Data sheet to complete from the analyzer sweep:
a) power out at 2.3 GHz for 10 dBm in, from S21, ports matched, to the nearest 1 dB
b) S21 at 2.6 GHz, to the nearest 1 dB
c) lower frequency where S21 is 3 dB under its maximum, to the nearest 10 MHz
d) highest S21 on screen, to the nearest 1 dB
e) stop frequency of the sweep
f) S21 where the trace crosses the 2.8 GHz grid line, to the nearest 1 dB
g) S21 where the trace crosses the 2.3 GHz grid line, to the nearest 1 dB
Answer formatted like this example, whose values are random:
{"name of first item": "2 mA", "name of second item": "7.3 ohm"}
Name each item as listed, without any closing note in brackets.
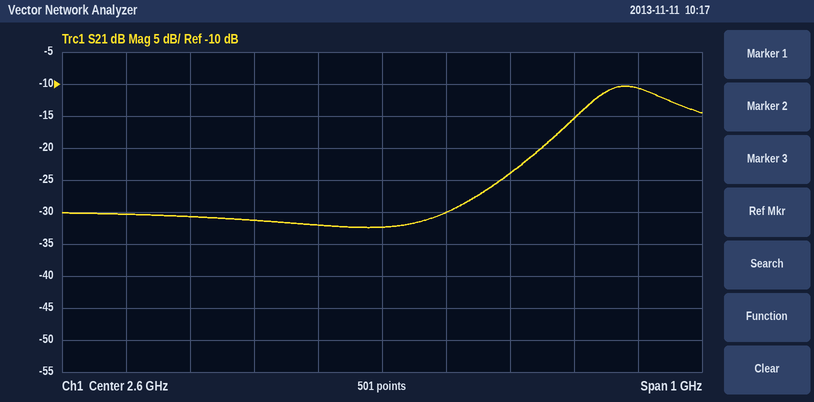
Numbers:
{"power out at 2.3 GHz for 10 dBm in, from S21, ports matched, to the nearest 1 dB": "-21 dBm", "S21 at 2.6 GHz, to the nearest 1 dB": "-32 dB", "lower frequency where S21 is 3 dB under its maximum, to the nearest 10 MHz": "2.92 GHz", "highest S21 on screen, to the nearest 1 dB": "-10 dB", "stop frequency of the sweep": "3.1 GHz", "S21 where the trace crosses the 2.8 GHz grid line, to the nearest 1 dB": "-24 dB", "S21 where the trace crosses the 2.3 GHz grid line, to the nearest 1 dB": "-31 dB"}
